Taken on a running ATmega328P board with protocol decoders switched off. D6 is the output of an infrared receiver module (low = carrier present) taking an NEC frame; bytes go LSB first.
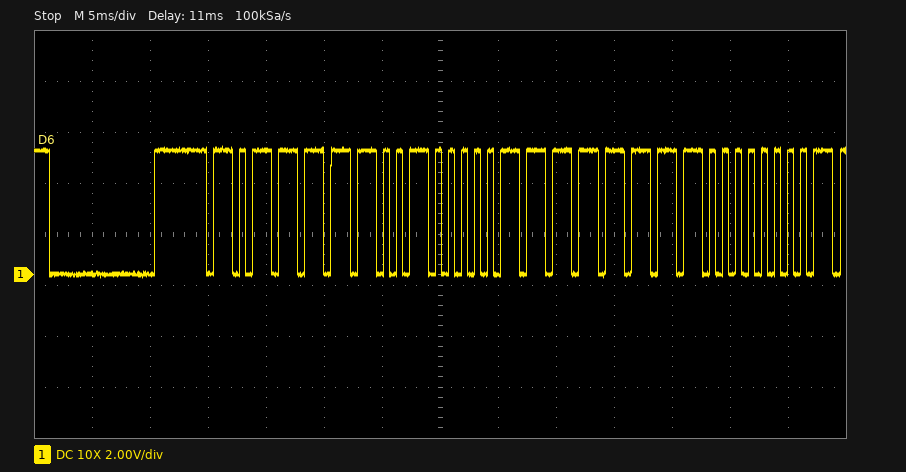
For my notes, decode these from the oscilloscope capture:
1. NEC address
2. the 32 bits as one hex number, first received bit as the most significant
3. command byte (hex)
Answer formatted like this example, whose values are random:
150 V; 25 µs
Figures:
0x7D; 0xBE41FE01; 0x7F
